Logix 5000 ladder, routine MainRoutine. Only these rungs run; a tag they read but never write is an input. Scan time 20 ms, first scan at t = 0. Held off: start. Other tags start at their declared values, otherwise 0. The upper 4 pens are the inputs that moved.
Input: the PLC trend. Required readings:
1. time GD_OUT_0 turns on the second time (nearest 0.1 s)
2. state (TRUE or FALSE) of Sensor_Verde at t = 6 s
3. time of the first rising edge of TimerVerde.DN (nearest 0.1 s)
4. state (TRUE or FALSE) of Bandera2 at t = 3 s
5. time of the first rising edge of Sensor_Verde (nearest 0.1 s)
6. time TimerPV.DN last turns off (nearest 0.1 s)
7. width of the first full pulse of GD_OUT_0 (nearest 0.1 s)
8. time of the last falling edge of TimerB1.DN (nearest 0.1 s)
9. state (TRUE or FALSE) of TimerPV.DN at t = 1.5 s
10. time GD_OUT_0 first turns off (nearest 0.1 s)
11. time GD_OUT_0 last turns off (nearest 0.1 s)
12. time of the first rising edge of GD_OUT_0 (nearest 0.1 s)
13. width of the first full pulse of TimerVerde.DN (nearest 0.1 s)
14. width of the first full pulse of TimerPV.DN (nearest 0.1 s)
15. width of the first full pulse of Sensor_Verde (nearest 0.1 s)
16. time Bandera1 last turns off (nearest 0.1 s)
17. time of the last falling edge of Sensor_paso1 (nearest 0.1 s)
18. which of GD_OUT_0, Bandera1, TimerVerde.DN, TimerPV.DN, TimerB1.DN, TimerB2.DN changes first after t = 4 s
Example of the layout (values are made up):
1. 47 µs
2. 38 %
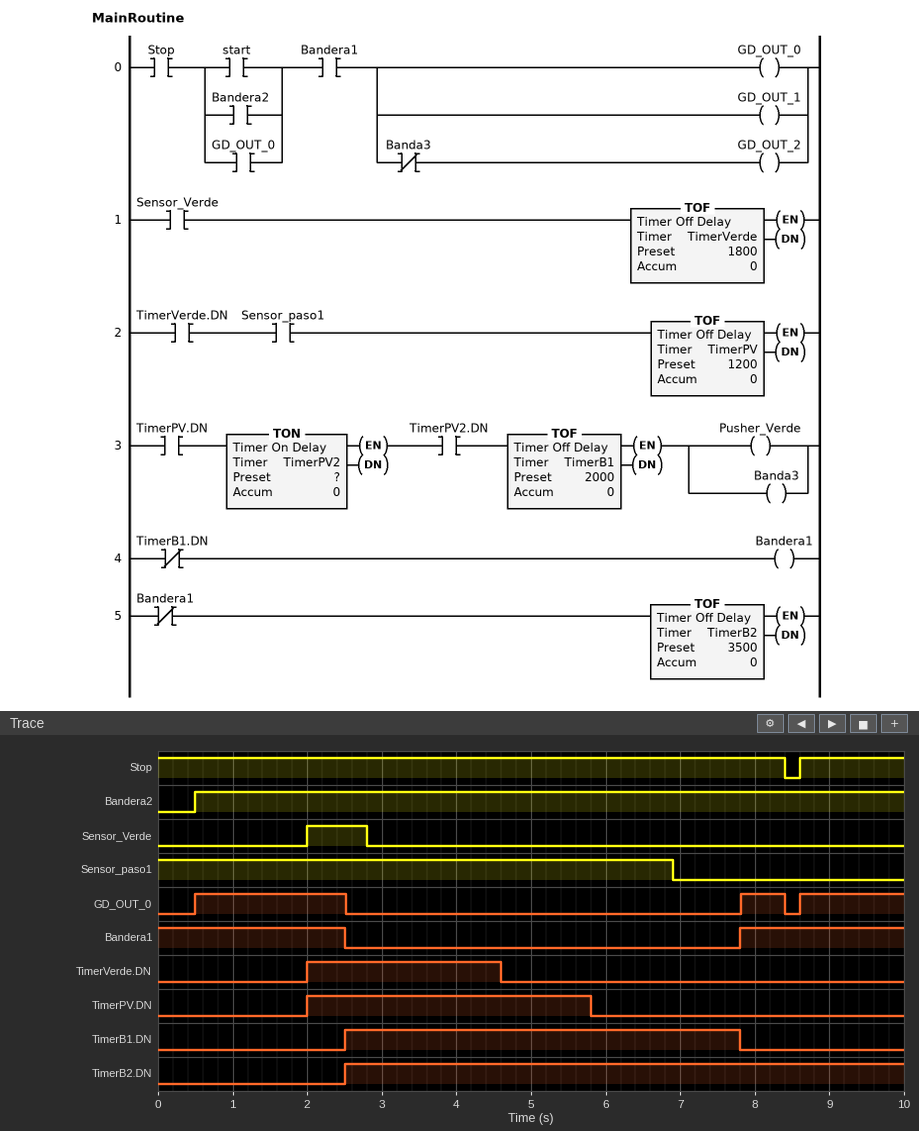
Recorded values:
1. 7.8 s
2. FALSE
3. 2.0 s
4. TRUE
5. 2.0 s
6. 5.8 s
7. 2.0 s
8. 7.8 s
9. FALSE
10. 2.5 s
11. 8.4 s
12. 0.5 s
13. 2.6 s
14. 3.8 s
15. 0.8 s
16. 2.5 s
17. 6.9 s
18. TimerVerde.DN
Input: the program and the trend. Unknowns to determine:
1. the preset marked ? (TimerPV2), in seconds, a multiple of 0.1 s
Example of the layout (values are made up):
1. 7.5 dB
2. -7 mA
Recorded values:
1. 0.5 s
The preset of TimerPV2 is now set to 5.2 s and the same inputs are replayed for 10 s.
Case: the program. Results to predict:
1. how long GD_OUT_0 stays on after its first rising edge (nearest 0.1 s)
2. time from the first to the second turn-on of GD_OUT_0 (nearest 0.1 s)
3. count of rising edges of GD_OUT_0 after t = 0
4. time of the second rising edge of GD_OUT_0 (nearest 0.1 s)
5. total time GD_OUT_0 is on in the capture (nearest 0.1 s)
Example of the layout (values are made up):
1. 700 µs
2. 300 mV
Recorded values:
1. 7.9 s
2. 8.1 s
3. 2
4. 8.6 s
5. 9.3 s
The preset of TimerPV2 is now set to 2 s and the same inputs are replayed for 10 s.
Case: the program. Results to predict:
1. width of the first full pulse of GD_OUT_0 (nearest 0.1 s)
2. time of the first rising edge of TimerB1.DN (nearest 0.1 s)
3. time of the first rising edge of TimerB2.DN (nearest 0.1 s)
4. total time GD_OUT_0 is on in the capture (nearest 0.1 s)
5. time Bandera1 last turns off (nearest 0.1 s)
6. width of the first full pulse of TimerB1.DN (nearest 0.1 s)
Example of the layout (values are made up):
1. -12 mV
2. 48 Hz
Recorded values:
1. 3.5 s
2. 4.0 s
3. 4.0 s
4. 5.5 s
5. 4.0 s
6. 3.8 s
